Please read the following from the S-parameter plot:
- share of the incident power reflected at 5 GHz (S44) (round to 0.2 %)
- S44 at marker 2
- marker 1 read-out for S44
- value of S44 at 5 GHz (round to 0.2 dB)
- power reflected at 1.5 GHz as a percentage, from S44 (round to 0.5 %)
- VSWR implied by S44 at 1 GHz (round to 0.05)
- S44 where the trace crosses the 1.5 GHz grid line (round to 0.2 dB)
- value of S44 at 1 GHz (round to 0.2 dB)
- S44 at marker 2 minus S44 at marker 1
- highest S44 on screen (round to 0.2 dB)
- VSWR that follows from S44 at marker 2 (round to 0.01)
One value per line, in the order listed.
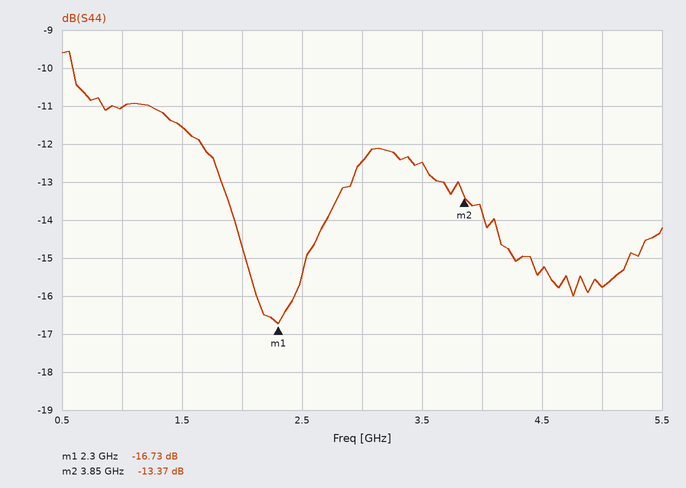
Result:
2.6 %
-13.37 dB
-16.73 dB
-15.8 dB
7.0 %
1.80
-11.6 dB
-11.0 dB
3.36 dB
-9.6 dB
1.55
